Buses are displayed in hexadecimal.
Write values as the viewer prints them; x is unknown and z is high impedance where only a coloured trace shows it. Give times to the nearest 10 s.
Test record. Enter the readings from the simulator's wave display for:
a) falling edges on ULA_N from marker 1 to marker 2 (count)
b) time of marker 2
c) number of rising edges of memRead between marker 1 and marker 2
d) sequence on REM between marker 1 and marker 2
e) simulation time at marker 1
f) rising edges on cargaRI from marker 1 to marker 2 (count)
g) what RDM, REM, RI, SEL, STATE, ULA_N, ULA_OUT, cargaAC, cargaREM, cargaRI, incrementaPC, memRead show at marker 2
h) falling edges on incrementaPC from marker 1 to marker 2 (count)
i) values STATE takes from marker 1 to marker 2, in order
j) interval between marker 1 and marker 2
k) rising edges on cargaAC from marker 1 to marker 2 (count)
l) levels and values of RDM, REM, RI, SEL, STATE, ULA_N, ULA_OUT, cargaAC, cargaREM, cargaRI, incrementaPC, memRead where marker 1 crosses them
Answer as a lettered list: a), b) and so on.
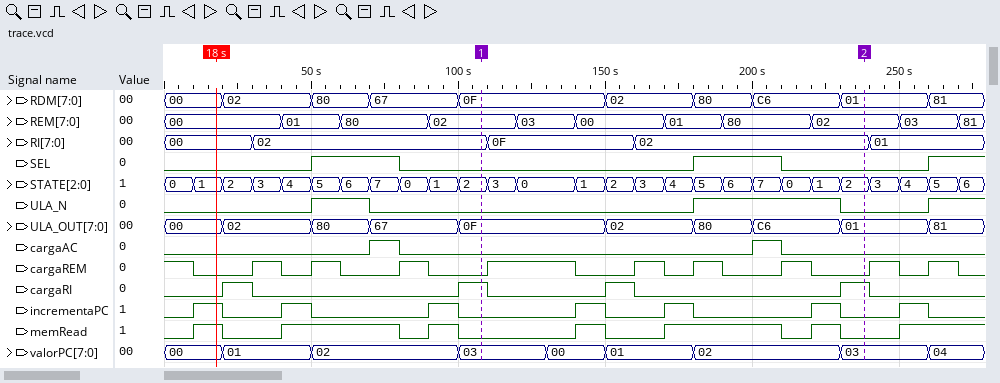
a) 1
b) 240 s
c) 3
d) 02, 03, 00, 01, 80, 02
e) 110 s
f) 2
g) RDM=01, REM=02, RI=02, SEL=0, STATE=2, ULA_N=0, ULA_OUT=01, cargaAC=0, cargaREM=0, cargaRI=1, incrementaPC=0, memRead=0
h) 3
i) 2, 3, 0, 1, 2, 3, 4, 5, 6, 7, 0, 1, 2
j) 130 s
k) 1
l) RDM=0F, REM=02, RI=02, SEL=0, STATE=2, ULA_N=0, ULA_OUT=0F, cargaAC=0, cargaREM=0, cargaRI=1, incrementaPC=0, memRead=0
